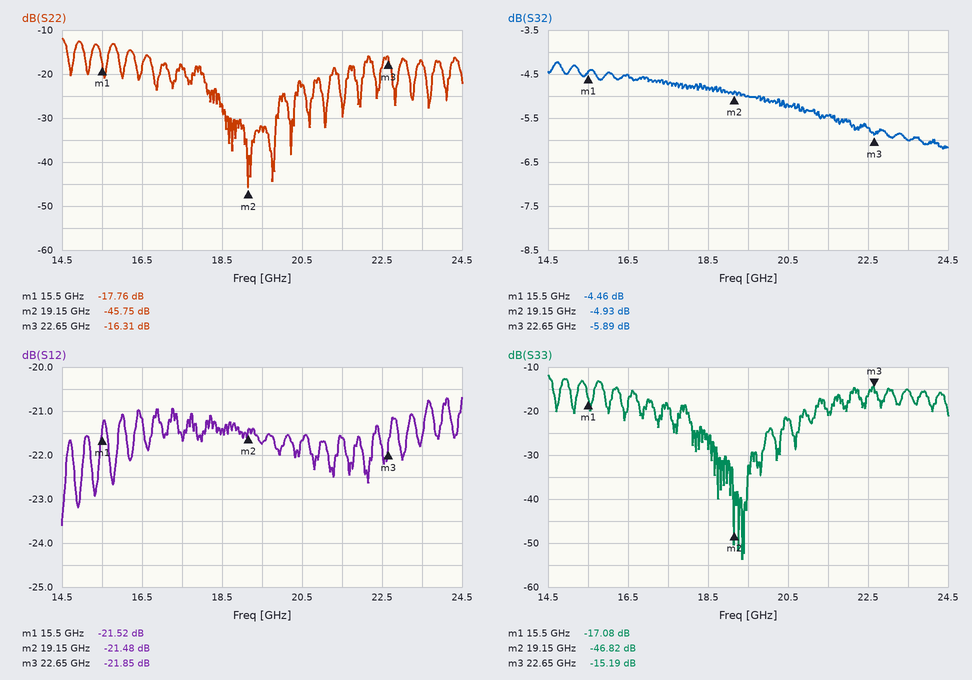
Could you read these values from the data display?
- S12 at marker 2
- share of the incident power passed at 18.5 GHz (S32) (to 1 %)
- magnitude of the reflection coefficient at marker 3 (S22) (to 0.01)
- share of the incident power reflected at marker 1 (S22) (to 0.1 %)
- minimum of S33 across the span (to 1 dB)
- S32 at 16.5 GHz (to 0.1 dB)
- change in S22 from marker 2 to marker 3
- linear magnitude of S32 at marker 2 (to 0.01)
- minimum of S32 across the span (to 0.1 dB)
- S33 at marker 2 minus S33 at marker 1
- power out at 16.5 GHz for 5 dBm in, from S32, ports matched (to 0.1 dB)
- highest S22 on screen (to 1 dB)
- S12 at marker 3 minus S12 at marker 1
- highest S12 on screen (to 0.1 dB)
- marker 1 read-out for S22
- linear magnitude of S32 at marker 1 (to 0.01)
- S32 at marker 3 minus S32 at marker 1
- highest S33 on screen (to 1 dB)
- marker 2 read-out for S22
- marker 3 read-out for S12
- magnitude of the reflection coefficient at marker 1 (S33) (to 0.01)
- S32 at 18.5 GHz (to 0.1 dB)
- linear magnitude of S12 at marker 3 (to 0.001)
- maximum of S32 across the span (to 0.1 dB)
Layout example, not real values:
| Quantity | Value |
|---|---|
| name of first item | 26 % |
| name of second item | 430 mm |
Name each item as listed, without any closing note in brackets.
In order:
| Quantity | Value |
|---|---|
| S12 at marker 2 | -21.48 dB |
| share of the incident power passed at 18.5 GHz (S32) | 33 % |
| magnitude of the reflection coefficient at marker 3 (S22) | 0.15 |
| share of the incident power reflected at marker 1 (S22) | 1.7 % |
| minimum of S33 across the span | -54 dB |
| S32 at 16.5 GHz | -4.5 dB |
| change in S22 from marker 2 to marker 3 | 29.44 dB |
| linear magnitude of S32 at marker 2 | 0.57 |
| minimum of S32 across the span | -6.2 dB |
| S33 at marker 2 minus S33 at marker 1 | -29.74 dB |
| power out at 16.5 GHz for 5 dBm in, from S32, ports matched | 0.5 dBm |
| highest S22 on screen | -12 dB |
| S12 at marker 3 minus S12 at marker 1 | -0.33 dB |
| highest S12 on screen | -20.7 dB |
| marker 1 read-out for S22 | -17.76 dB |
| linear magnitude of S32 at marker 1 | 0.60 |
| S32 at marker 3 minus S32 at marker 1 | -1.43 dB |
| highest S33 on screen | -12 dB |
| marker 2 read-out for S22 | -45.75 dB |
| marker 3 read-out for S12 | -21.85 dB |
| magnitude of the reflection coefficient at marker 1 (S33) | 0.14 |
| S32 at 18.5 GHz | -4.8 dB |
| linear magnitude of S12 at marker 3 | 0.081 |
| maximum of S32 across the span | -4.2 dB |
